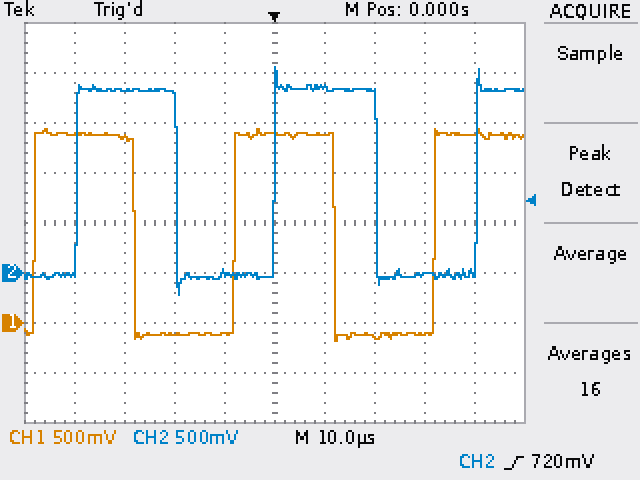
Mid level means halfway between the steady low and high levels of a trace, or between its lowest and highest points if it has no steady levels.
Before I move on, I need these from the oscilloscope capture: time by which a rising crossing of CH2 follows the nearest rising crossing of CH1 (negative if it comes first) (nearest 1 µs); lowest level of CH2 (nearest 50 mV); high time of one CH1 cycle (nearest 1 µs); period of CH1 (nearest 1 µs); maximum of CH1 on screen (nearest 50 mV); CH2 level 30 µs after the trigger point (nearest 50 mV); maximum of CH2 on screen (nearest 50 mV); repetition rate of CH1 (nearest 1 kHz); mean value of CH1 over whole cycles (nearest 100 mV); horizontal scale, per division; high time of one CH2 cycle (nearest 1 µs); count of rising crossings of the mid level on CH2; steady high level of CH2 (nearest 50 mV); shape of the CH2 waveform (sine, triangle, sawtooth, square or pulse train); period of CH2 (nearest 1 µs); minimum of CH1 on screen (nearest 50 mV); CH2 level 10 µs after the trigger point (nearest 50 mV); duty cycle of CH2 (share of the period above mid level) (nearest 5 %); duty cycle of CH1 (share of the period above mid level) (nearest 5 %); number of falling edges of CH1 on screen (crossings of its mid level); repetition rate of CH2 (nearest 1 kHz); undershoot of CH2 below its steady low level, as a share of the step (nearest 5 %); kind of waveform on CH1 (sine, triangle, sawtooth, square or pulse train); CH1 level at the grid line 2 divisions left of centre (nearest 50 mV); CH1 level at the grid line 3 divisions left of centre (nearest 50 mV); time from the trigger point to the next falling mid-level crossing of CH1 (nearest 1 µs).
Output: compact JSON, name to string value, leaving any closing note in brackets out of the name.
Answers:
{"time by which a rising crossing of CH2 follows the nearest rising crossing of CH1 (negative if it comes first)": "+8 µs", "lowest level of CH2": "-200 mV", "high time of one CH1 cycle": "20 µs", "period of CH1": "40 µs", "maximum of CH1 on screen": "1.95 V", "CH2 level 30 µs after the trigger point": "0 mV", "maximum of CH2 on screen": "2.05 V", "repetition rate of CH1": "25 kHz", "mean value of CH1 over whole cycles": "900 mV", "horizontal scale, per division": "10 µs", "high time of one CH2 cycle": "20 µs", "count of rising crossings of the mid level on CH2": "3", "steady high level of CH2": "1.85 V", "shape of the CH2 waveform": "square", "period of CH2": "40 µs", "minimum of CH1 on screen": "-200 mV", "CH2 level 10 µs after the trigger point": "1.85 V", "duty cycle of CH2 (share of the period above mid level)": "50 %", "duty cycle of CH1 (share of the period above mid level)": "50 %", "number of falling edges of CH1 on screen": "2", "repetition rate of CH2": "25 kHz", "undershoot of CH2 below its steady low level, as a share of the step": "10 %", "kind of waveform on CH1": "square", "CH1 level at the grid line 2 divisions left of centre": "-100 mV", "CH1 level at the grid line 3 divisions left of centre": "1.85 V", "time from the trigger point to the next falling mid-level crossing of CH1": "12 µs"}
